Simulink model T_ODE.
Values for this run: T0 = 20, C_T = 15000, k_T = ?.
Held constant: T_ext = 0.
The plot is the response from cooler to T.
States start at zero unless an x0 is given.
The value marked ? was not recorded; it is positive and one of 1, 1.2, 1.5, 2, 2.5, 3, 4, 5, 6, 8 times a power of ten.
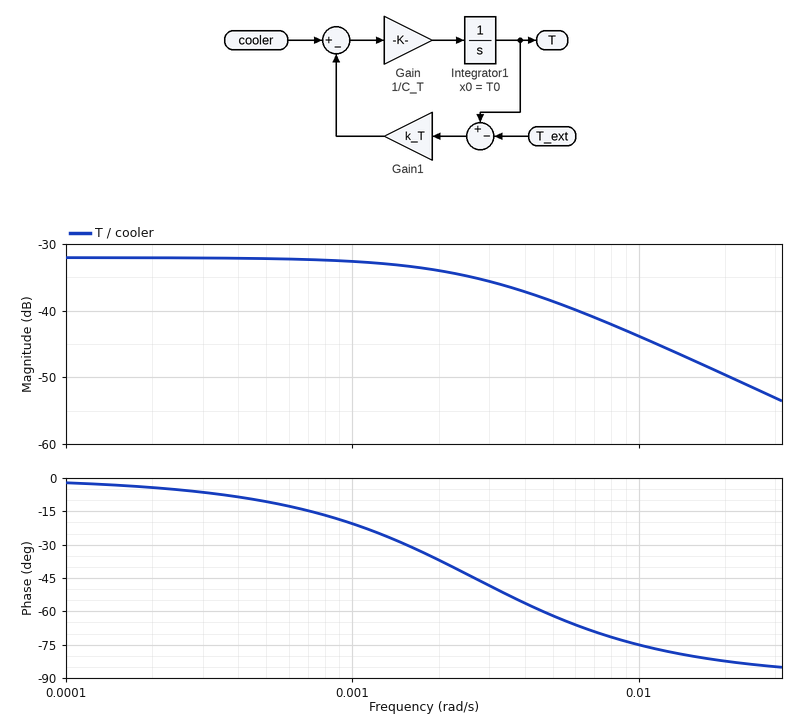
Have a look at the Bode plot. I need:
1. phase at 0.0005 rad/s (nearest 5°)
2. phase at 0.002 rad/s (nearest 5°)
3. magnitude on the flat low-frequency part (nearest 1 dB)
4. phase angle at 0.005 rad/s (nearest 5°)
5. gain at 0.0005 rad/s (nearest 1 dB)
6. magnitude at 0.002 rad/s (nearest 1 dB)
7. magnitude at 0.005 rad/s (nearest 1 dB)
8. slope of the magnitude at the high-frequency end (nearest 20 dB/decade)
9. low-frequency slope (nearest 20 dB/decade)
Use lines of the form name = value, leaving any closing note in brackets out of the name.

phase at 0.0005 rad/s = -10°
phase at 0.002 rad/s = -35°
magnitude on the flat low-frequency part = -32 dB
phase angle at 0.005 rad/s = -60°
gain at 0.0005 rad/s = -32 dB
magnitude at 0.002 rad/s = -34 dB
magnitude at 0.005 rad/s = -39 dB
slope of the magnitude at the high-frequency end = -20 dB/decade
low-frequency slope = 0 dB/decade
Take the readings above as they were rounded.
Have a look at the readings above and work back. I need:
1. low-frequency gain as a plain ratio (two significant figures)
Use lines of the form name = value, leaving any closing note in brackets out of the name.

low-frequency gain as a plain ratio = 0.025
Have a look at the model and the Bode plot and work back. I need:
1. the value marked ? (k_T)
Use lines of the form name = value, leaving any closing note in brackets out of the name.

the value marked ? = 40
